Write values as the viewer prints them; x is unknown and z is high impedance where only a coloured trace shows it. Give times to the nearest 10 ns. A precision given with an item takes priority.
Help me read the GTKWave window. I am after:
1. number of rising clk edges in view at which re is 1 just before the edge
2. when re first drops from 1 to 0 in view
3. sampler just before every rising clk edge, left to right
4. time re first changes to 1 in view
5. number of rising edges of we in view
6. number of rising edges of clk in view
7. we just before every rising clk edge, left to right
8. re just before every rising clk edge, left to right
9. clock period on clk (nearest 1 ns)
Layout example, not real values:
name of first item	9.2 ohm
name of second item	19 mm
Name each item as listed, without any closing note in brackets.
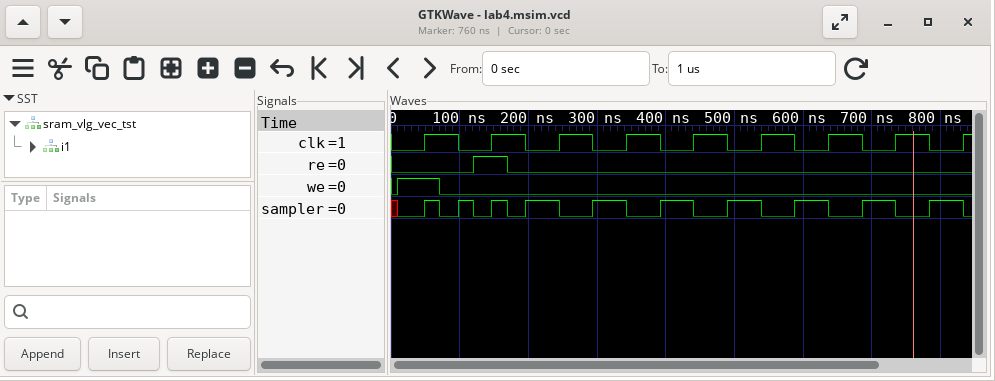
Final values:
number of rising clk edges in view at which re is 1 just before the edge	1
when re first drops from 1 to 0 in view	170 ns
sampler just before every rising clk edge, left to right	0 0 1 1 1 1 1 1 1
time re first changes to 1 in view	120 ns
number of rising edges of we in view	1
number of rising edges of clk in view	9
we just before every rising clk edge, left to right	1 0 0 0 0 0 0 0 0
re just before every rising clk edge, left to right	0 1 0 0 0 0 0 0 0
clock period on clk	98 ns
